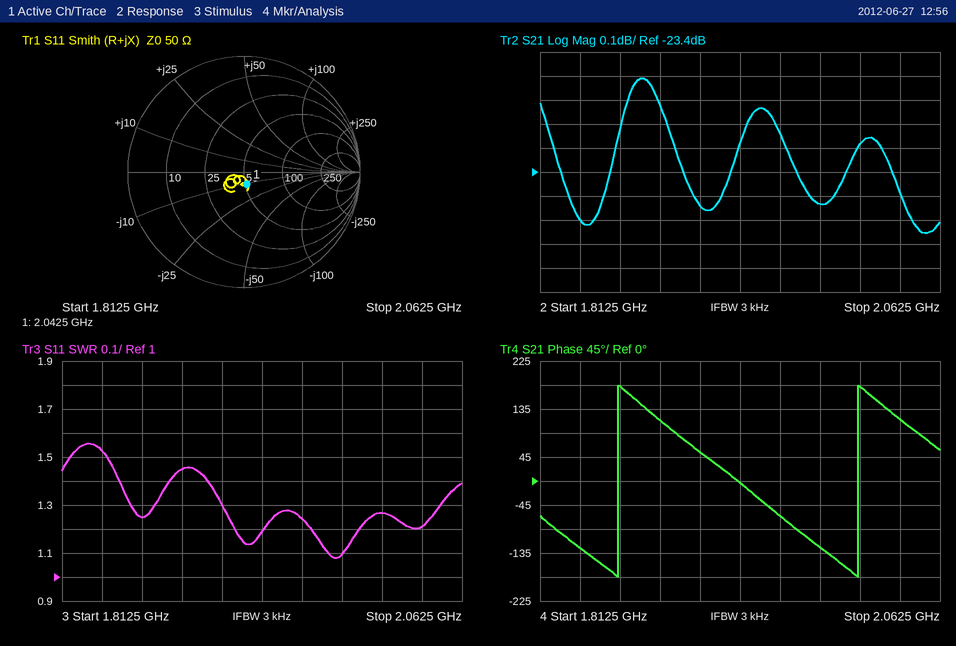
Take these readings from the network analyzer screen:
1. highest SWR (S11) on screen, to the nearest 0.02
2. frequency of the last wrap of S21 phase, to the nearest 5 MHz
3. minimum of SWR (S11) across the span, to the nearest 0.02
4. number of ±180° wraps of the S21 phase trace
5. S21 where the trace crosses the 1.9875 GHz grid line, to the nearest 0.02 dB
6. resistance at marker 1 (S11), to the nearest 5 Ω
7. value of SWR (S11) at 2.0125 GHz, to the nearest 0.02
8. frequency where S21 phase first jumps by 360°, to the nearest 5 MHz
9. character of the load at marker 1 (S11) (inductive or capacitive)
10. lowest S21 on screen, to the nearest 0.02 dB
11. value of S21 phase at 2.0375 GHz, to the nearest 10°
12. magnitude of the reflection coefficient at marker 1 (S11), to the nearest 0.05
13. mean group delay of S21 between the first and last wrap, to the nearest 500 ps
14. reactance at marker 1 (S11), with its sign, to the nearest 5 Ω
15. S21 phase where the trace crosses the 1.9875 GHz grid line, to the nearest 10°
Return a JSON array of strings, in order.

["1.56", "2.010 GHz", "1.08", "2", "-23.54 dB", "50 Ω", "1.26", "1.860 GHz", "capacitive", "-23.66 dB", "120°", "0.10", "6.5 ns", "-10 Ω", "-120°"]
